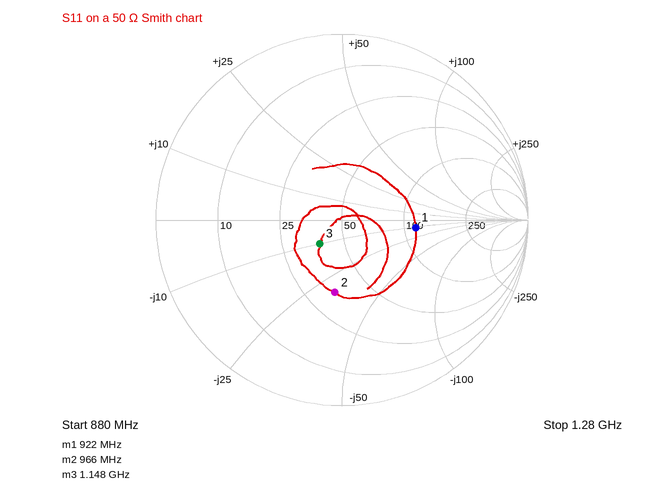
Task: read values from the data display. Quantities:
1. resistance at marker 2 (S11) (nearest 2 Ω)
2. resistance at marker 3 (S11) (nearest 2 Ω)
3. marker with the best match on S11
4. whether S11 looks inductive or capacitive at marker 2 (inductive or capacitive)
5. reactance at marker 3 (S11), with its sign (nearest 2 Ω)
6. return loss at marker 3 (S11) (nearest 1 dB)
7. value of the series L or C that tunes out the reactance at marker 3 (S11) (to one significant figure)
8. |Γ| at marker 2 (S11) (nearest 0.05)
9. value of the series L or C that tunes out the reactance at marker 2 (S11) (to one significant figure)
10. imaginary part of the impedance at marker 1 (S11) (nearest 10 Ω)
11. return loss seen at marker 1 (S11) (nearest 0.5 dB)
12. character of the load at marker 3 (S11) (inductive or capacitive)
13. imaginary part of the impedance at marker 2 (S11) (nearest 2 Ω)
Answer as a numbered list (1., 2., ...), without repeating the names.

1. 34 Ω
2. 38 Ω
3. marker 3
4. capacitive
5. -10 Ω
6. 15 dB
7. 1 nH
8. 0.40
9. 5 nH
10. -10 Ω
11. 8.0 dB
12. capacitive
13. -32 Ω
